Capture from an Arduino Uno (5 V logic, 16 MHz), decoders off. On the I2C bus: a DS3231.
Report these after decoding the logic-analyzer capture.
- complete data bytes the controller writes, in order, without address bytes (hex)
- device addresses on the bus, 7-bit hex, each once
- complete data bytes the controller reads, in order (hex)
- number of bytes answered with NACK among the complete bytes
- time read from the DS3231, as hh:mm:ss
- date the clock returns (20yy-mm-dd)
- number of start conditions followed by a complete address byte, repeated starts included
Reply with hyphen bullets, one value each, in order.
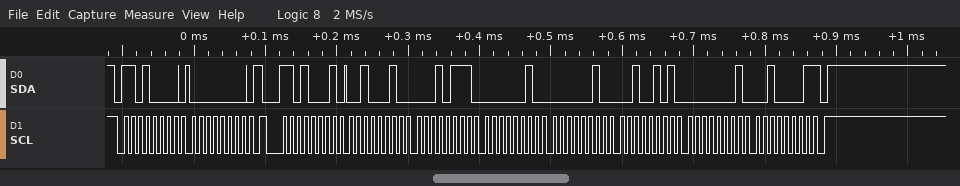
- 00
- 0x68
- 22 17 02 02 25 01 21
- 1
- 02:17:22
- 2021-01-25
- 2
